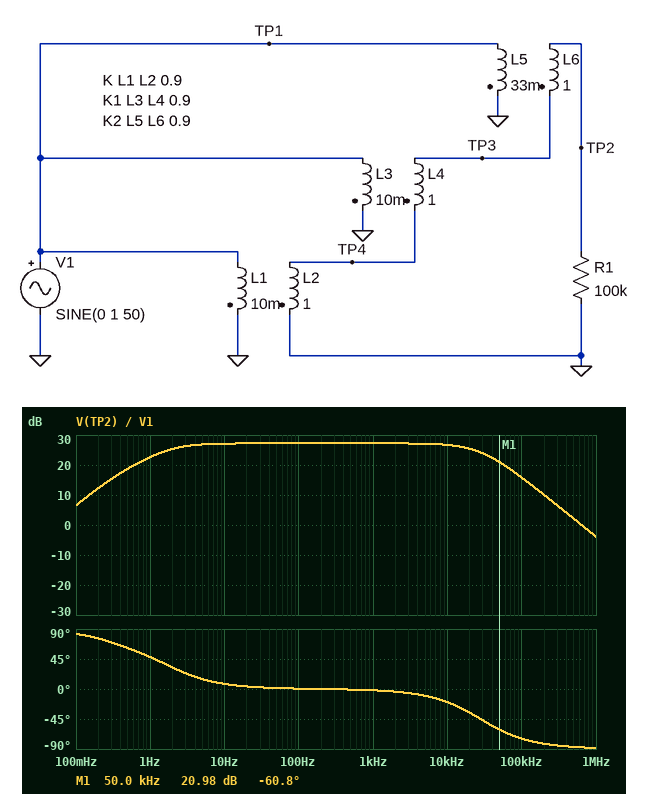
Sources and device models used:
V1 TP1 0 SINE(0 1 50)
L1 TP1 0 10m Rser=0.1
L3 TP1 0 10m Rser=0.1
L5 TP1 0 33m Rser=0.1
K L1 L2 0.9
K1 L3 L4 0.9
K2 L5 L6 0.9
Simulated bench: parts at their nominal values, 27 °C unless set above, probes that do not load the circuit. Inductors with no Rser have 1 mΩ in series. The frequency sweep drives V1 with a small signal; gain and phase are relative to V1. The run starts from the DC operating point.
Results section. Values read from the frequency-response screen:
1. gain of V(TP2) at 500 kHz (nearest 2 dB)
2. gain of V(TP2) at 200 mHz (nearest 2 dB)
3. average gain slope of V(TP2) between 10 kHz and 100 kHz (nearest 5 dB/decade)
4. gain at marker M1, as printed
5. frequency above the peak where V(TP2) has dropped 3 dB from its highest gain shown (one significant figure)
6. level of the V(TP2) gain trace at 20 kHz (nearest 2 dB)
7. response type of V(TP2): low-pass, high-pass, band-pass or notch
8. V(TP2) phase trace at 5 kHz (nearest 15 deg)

2 dB
12 dB
-10 dB/decade
20.98 dB
30 kHz
26 dB
band-pass
-15 deg
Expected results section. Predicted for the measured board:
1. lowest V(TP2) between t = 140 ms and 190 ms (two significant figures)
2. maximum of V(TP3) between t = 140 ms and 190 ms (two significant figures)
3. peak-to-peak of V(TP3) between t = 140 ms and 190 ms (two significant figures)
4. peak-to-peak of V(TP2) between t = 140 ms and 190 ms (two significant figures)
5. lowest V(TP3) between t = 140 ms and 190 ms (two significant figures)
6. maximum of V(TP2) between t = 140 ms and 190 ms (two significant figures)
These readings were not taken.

-23 V
18 V
36 V
46 V
-18 V
23 V
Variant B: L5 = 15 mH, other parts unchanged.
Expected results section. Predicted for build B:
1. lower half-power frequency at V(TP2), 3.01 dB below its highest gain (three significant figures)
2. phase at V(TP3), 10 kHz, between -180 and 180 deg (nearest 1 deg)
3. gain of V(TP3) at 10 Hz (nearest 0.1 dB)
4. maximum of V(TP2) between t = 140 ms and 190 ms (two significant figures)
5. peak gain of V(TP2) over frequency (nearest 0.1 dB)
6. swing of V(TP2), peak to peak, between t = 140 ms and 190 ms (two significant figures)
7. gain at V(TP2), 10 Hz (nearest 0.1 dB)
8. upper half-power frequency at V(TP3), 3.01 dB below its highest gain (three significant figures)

1.44 Hz
-18 deg
25.0 dB
25 V
28.1 dB
51 V
28.0 dB
28.0 kHz
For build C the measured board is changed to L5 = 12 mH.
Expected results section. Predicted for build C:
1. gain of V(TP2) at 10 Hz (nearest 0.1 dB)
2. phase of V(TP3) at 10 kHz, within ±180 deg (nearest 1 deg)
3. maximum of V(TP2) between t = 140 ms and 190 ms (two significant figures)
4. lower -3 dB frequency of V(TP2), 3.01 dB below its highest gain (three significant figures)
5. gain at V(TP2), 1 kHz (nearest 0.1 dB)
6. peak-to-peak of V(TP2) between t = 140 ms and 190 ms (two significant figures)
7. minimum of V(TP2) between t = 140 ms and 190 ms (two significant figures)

28.3 dB
-19 deg
26 V
1.51 Hz
28.4 dB
52 V
-26 V
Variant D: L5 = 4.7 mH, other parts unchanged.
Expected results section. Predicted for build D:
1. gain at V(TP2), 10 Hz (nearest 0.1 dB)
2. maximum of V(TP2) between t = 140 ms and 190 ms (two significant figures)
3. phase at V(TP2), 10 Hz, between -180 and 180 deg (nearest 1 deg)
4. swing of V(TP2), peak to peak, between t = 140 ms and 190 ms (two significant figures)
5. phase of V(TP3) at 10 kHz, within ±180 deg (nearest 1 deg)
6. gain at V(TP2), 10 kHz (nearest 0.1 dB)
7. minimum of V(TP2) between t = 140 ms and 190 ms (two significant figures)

29.6 dB
31 V
13 deg
62 V
-23 deg
29.3 dB
-31 V
